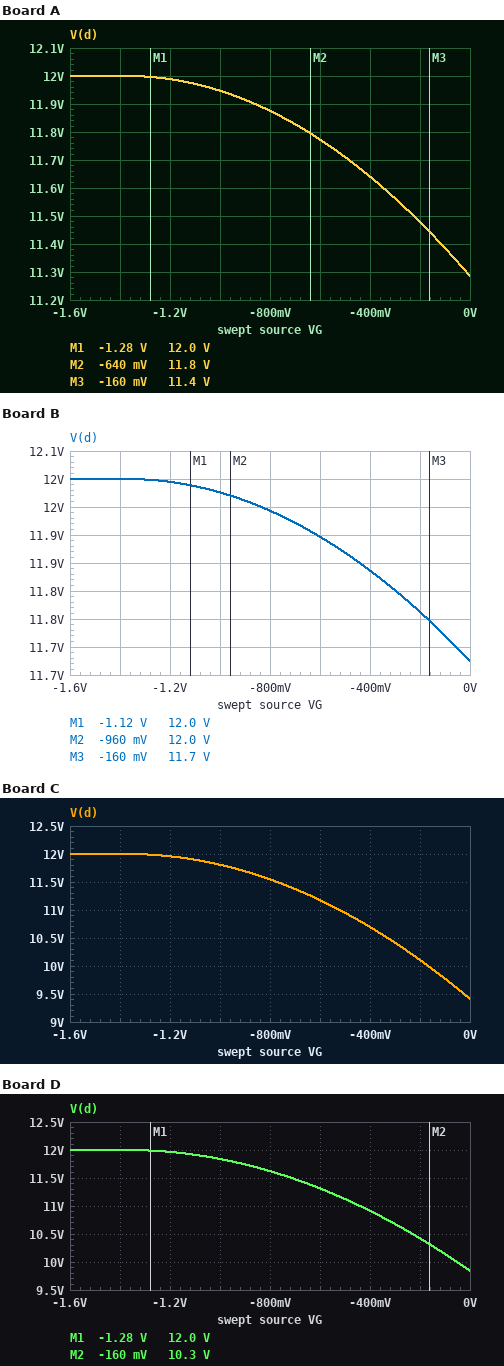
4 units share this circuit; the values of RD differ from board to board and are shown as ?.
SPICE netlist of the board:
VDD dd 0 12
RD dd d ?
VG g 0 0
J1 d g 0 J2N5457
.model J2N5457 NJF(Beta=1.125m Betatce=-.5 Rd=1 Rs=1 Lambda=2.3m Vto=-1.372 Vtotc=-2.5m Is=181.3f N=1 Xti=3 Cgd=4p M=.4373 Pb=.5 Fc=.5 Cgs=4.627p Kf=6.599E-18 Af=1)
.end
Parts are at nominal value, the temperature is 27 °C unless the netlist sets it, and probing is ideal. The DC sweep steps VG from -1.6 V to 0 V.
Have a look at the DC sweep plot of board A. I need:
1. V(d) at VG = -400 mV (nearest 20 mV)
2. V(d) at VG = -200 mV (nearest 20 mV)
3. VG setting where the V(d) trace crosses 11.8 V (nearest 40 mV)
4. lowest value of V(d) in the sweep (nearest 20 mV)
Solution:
11.64 V
11.48 V
-640 mV
11.28 V
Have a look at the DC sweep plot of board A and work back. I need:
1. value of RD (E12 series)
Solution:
330 Ω
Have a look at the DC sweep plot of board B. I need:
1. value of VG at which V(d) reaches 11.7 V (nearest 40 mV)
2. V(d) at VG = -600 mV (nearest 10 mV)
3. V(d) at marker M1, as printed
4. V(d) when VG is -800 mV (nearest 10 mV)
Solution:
-40 mV
11.90 V
12.0 V
11.94 V
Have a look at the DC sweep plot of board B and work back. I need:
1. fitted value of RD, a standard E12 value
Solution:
150 Ω
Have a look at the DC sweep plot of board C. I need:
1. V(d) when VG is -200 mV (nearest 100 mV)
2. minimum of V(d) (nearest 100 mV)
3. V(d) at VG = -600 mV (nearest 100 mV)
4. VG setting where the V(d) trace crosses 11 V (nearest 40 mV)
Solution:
10.1 V
9.4 V
11.2 V
-520 mV
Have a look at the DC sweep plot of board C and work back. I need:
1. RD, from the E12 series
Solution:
1.2 kΩ
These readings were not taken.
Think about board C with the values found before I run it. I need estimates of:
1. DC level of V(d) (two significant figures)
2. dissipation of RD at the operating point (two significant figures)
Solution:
9.4 V
5.6 mW
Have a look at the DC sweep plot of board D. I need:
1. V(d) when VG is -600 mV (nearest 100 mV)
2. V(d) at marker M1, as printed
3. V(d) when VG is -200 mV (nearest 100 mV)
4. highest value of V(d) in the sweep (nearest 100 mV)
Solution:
11.3 V
12.0 V
10.4 V
12.0 V
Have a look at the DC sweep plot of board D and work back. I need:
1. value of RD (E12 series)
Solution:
1 kΩ
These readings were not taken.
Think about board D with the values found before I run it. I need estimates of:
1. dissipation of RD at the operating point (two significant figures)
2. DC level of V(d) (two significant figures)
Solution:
4.7 mW
9.8 V
